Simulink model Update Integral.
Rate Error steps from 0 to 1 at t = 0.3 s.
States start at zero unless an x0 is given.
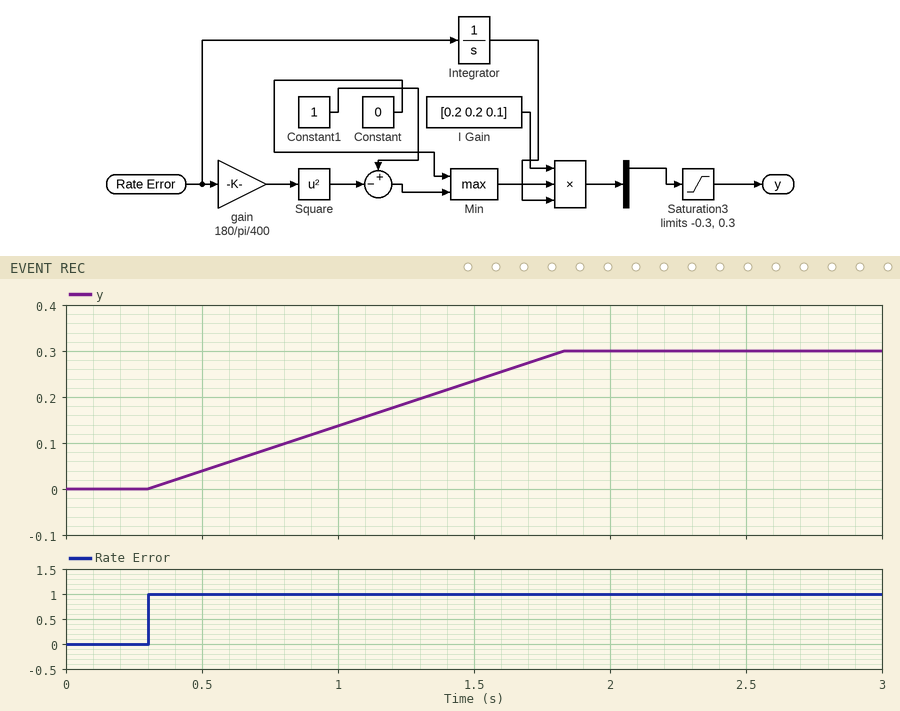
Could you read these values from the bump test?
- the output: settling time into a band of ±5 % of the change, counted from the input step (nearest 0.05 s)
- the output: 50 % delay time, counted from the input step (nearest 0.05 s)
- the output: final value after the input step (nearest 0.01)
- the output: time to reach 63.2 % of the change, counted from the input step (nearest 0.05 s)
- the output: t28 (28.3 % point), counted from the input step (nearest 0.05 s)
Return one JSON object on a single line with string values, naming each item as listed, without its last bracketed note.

{"the output: settling time into a band of ±5 % of the change, counted from the input step": "1.45 s", "the output: 50 % delay time, counted from the input step": "0.75 s", "the output: final value after the input step": "0.30", "the output: time to reach 63.2 % of the change, counted from the input step": "0.95 s", "the output: t28 (28.3 % point), counted from the input step": "0.45 s"}
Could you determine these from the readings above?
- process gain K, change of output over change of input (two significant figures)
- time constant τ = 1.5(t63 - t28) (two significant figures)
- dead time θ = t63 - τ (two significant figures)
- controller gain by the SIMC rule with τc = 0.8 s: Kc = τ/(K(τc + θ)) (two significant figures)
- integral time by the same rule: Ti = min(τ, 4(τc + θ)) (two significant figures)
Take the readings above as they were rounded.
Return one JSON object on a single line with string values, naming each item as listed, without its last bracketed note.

{"process gain K, change of output over change of input": "0.30", "time constant τ = 1.5(t63 - t28)": "0.75 s", "dead time θ = t63 - τ": "0.20 s", "controller gain by the SIMC rule with τc = 0.8 s: Kc = τ/(K(τc + θ))": "2.5", "integral time by the same rule: Ti = min(τ, 4(τc + θ))": "0.75 s"}
